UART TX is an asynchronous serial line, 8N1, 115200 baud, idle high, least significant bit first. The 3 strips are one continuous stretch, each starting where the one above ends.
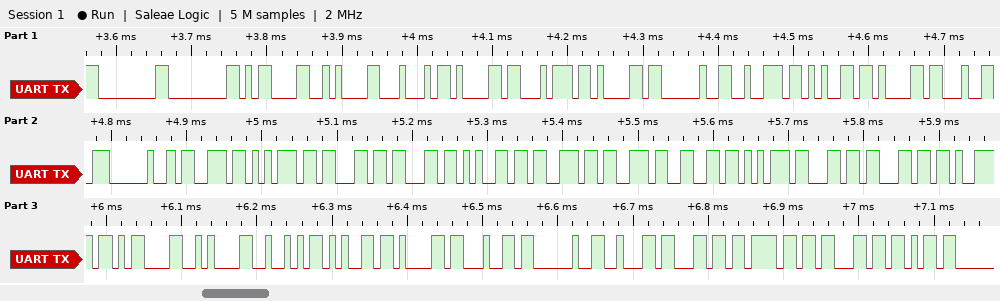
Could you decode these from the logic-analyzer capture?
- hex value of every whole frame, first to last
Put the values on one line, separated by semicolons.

00 00 0D 0A 44 61 74 61 20 72 65 61 64 20 73 75 63 63 65 73 73 66 75 6C 6C 79 0D 0A 52 65 61 64 20 62 6C 6F 63 6B
